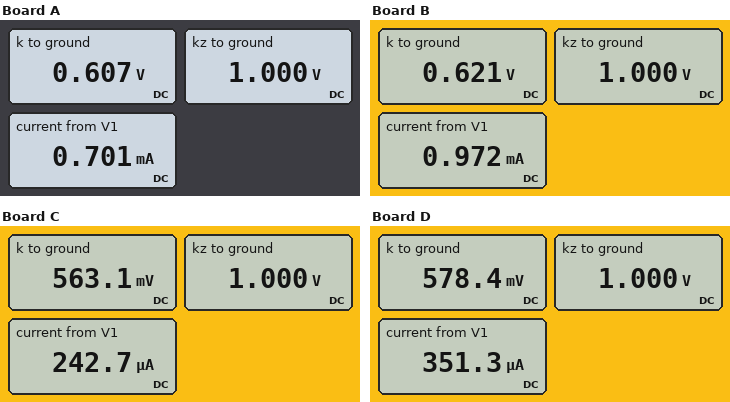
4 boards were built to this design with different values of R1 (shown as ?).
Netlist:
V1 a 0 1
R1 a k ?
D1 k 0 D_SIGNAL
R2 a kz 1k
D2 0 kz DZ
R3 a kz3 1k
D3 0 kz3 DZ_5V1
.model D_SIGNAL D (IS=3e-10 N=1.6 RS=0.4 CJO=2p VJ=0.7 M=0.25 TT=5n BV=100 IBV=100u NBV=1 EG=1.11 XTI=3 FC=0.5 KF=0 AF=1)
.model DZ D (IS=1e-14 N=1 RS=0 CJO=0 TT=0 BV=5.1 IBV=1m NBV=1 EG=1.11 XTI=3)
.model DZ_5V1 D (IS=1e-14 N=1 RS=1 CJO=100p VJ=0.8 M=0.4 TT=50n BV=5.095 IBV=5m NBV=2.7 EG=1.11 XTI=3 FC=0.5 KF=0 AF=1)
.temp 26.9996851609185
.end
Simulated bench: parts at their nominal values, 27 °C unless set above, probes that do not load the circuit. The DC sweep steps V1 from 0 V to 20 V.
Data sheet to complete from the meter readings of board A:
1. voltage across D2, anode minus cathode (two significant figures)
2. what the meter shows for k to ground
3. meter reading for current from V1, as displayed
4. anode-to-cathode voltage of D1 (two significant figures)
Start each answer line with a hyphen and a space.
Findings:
- -1.0 V
- 0.607 V
- 0.701 mA
- 610 mV
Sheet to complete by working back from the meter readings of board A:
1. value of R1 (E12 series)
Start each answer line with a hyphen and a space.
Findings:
- 560 Ω
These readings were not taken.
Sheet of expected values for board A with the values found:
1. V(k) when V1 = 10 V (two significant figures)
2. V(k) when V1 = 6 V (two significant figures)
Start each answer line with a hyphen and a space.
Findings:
- 740 mV
- 720 mV
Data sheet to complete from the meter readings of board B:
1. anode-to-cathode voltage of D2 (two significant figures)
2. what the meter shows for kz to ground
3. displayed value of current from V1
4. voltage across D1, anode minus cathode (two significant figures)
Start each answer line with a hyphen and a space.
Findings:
- -1.0 V
- 1.000 V
- 0.972 mA
- 620 mV
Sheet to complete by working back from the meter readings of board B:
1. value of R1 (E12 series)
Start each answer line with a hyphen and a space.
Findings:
- 390 Ω
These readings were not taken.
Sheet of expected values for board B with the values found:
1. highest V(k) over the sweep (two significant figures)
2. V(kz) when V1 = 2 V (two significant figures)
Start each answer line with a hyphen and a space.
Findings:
- 800 mV
- 2.0 V
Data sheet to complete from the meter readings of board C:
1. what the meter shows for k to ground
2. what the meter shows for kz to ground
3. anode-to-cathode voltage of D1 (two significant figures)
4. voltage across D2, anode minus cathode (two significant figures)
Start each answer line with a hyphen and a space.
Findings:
- 563.1 mV
- 1.000 V
- 560 mV
- -1.0 V
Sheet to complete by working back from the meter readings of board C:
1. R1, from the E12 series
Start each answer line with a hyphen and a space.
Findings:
- 1.8 kΩ
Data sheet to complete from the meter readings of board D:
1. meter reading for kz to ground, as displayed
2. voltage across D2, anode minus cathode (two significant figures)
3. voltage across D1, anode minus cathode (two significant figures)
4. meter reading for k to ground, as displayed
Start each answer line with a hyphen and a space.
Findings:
- 1.000 V
- -1.0 V
- 580 mV
- 578.4 mV
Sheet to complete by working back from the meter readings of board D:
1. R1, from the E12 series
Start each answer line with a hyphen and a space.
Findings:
- 1.2 kΩ
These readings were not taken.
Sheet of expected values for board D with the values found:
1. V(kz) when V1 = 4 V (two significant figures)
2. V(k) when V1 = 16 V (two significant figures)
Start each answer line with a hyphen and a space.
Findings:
- 4.0 V
- 730 mV
